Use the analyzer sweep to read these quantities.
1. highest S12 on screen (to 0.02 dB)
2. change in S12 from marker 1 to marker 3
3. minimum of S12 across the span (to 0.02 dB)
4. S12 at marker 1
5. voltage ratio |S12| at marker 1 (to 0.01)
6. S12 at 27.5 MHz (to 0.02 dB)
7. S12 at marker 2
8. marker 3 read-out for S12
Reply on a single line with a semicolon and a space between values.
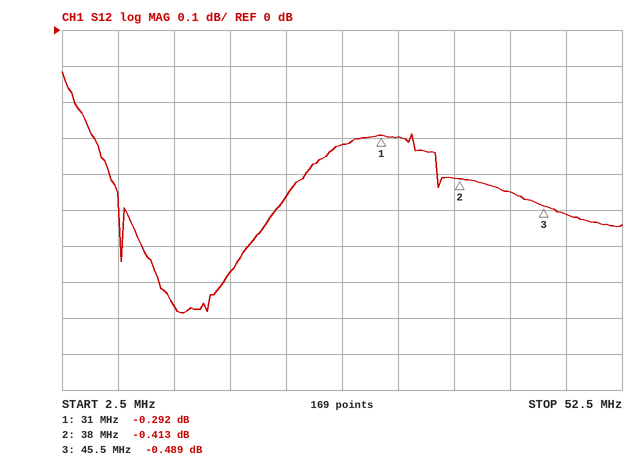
-0.12 dB; -0.197 dB; -0.78 dB; -0.292 dB; 0.97; -0.32 dB; -0.413 dB; -0.489 dB
